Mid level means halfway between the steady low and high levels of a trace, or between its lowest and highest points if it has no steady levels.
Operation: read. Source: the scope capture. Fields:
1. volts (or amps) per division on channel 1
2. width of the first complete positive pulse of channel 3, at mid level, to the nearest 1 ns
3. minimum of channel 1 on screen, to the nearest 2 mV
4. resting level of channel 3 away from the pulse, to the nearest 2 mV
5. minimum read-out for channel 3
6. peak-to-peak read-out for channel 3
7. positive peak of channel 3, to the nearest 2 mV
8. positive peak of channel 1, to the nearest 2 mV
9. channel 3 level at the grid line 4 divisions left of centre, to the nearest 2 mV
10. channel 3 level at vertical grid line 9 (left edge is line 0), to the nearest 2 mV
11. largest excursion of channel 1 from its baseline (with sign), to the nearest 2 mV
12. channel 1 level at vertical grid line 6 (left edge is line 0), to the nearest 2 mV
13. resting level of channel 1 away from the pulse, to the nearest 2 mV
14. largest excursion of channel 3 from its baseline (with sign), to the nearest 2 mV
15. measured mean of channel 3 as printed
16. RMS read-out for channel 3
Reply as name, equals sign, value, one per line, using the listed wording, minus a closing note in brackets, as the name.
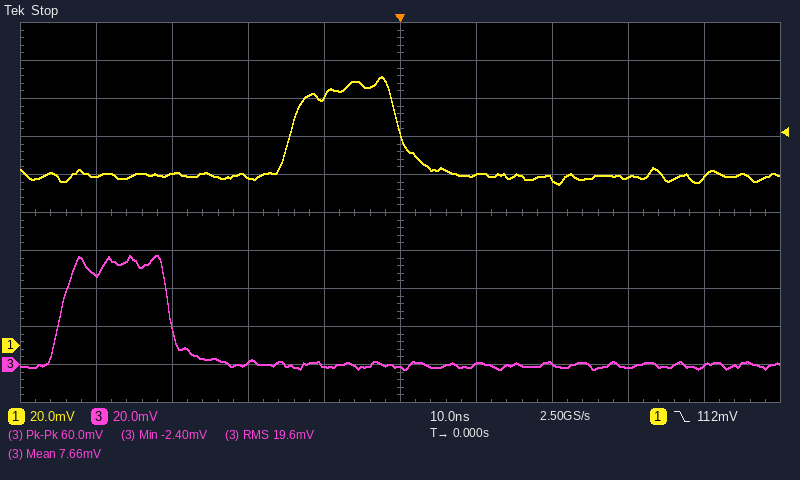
volts (or amps) per division on channel 1 = 20 mV
width of the first complete positive pulse of channel 3, at mid level, to the nearest 1 ns = 14 ns
minimum of channel 1 on screen, to the nearest 2 mV = 84 mV
resting level of channel 3 away from the pulse, to the nearest 2 mV = 0 mV
minimum read-out for channel 3 = -2.40 mV
peak-to-peak read-out for channel 3 = 60.0 mV
positive peak of channel 3, to the nearest 2 mV = 58 mV
positive peak of channel 1, to the nearest 2 mV = 142 mV
channel 3 level at the grid line 4 divisions left of centre, to the nearest 2 mV = 48 mV
channel 3 level at vertical grid line 9 (left edge is line 0), to the nearest 2 mV = 0 mV
largest excursion of channel 1 from its baseline (with sign), to the nearest 2 mV = +52 mV
channel 1 level at vertical grid line 6 (left edge is line 0), to the nearest 2 mV = 90 mV
resting level of channel 1 away from the pulse, to the nearest 2 mV = 90 mV
largest excursion of channel 3 from its baseline (with sign), to the nearest 2 mV = +58 mV
measured mean of channel 3 as printed = 7.66 mV
RMS read-out for channel 3 = 19.6 mV
